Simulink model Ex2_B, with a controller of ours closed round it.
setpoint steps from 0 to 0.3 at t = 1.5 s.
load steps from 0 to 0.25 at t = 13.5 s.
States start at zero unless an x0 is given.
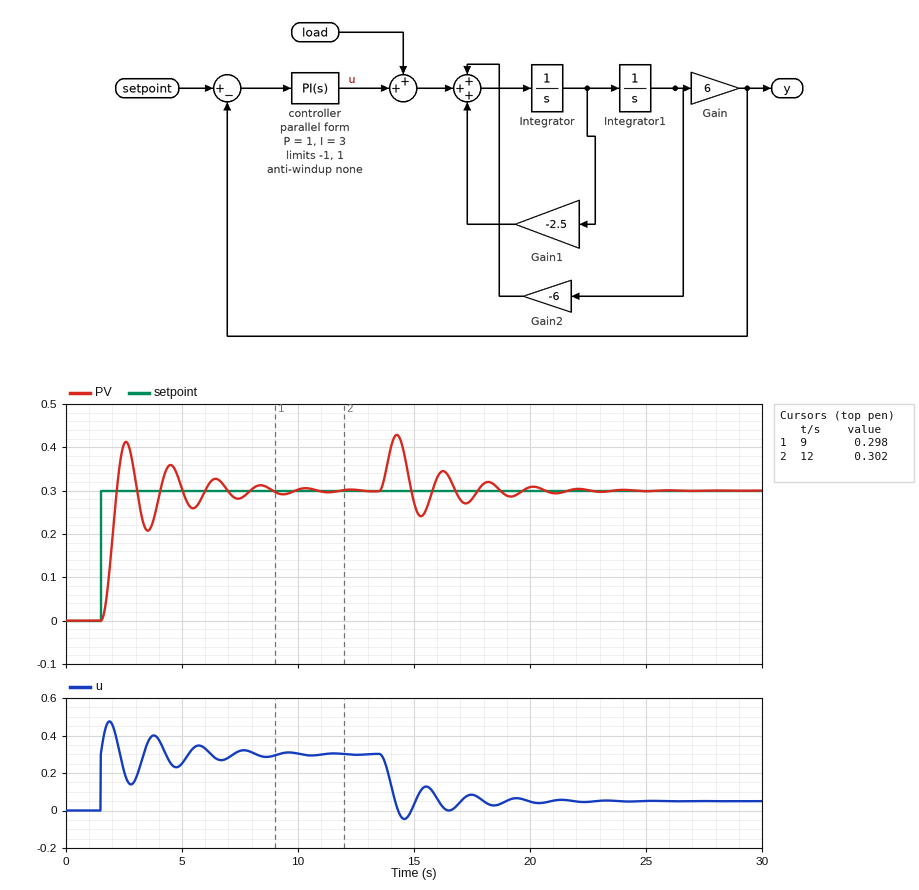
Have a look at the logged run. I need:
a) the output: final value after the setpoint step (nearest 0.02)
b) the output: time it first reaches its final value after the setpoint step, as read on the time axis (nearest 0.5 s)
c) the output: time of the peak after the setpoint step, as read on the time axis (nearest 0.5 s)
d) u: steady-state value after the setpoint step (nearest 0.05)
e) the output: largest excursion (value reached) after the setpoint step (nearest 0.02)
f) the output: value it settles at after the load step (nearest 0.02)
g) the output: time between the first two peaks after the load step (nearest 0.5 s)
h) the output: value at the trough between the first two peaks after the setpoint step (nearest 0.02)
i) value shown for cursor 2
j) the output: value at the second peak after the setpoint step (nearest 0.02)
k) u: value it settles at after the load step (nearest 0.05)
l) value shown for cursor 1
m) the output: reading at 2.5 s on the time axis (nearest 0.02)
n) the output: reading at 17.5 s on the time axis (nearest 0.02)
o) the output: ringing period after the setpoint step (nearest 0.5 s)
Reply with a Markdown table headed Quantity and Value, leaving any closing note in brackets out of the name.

| Quantity | Value |
|---|---|
| the output: final value after the setpoint step | 0.30 |
| the output: time it first reaches its final value after the setpoint step, as read on the time axis | 2.0 s |
| the output: time of the peak after the setpoint step, as read on the time axis | 2.5 s |
| u: steady-state value after the setpoint step | 0.30 |
| the output: largest excursion (value reached) after the setpoint step | 0.42 |
| the output: value it settles at after the load step | 0.30 |
| the output: time between the first two peaks after the load step | 2.0 s |
| the output: value at the trough between the first two peaks after the setpoint step | 0.20 |
| value shown for cursor 2 | 0.302 |
| the output: value at the second peak after the setpoint step | 0.36 |
| u: value it settles at after the load step | 0.05 |
| value shown for cursor 1 | 0.298 |
| the output: reading at 2.5 s on the time axis | 0.40 |
| the output: reading at 17.5 s on the time axis | 0.28 |
| the output: ringing period after the setpoint step | 2.0 s |
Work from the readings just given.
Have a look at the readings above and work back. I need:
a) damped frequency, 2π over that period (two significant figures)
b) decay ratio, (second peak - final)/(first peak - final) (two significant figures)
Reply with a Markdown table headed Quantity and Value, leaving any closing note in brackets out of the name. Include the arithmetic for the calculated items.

| Quantity | Value |
|---|---|
| damped frequency, 2π over that period | 2π / 2 = 3.1 rad/s |
| decay ratio, (second peak - final)/(first peak - final) | (0.36 - 0.3) / (0.42 - 0.3) = 0.50 |
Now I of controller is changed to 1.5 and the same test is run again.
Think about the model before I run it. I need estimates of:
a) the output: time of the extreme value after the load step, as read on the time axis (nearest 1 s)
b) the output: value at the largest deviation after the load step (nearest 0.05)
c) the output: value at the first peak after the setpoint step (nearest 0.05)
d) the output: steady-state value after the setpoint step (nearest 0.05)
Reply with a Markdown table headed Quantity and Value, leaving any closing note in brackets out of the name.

| Quantity | Value |
|---|---|
| the output: time of the extreme value after the load step, as read on the time axis | 14 s |
| the output: value at the largest deviation after the load step | 0.45 |
| the output: value at the first peak after the setpoint step | 0.30 |
| the output: steady-state value after the setpoint step | 0.30 |
